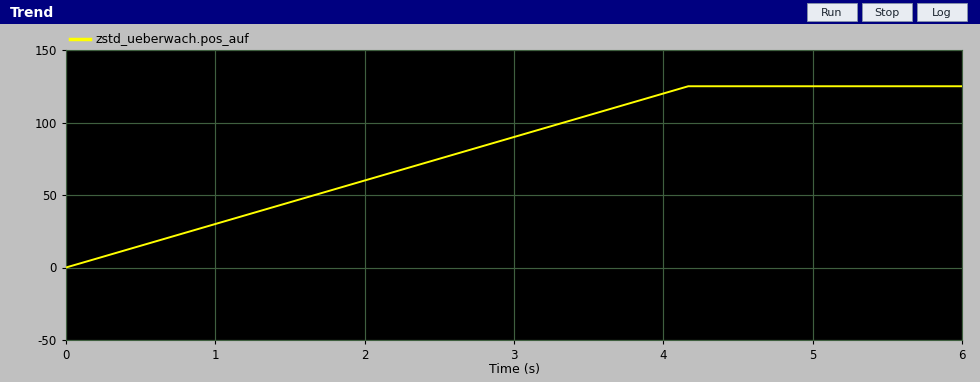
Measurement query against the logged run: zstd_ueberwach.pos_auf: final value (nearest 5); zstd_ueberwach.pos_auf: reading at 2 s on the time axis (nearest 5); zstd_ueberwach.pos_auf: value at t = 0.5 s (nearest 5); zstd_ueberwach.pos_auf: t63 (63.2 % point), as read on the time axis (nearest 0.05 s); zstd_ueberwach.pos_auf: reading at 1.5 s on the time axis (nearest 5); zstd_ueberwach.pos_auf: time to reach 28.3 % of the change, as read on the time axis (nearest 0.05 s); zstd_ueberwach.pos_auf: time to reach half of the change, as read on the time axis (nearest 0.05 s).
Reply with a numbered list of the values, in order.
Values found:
1. 125
2. 60
3. 15
4. 2.65 s
5. 45
6. 1.20 s
7. 2.10 s
